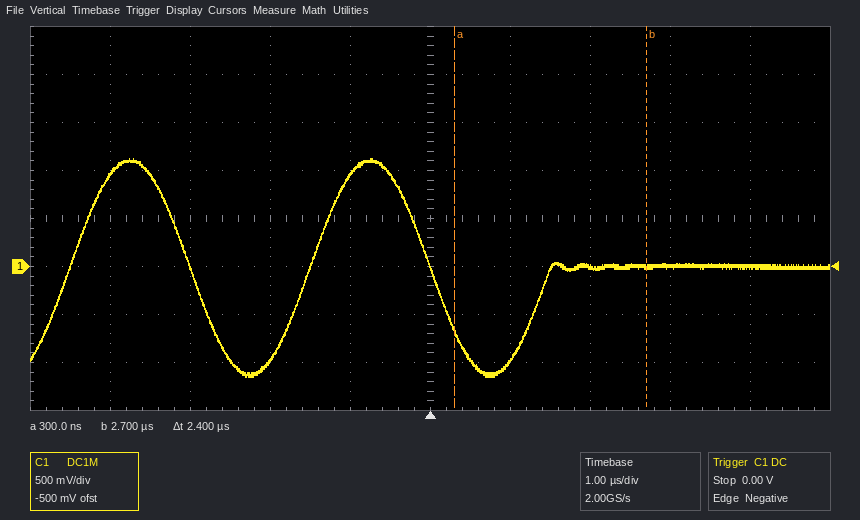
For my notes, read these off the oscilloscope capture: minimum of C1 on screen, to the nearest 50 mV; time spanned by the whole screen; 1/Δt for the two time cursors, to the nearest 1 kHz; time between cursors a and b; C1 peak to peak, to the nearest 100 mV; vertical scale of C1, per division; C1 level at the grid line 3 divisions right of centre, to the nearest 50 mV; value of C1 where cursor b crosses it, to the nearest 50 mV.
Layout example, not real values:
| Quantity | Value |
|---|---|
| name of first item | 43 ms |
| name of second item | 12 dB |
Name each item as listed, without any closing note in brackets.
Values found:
| Quantity | Value |
|---|---|
| minimum of C1 on screen, to the nearest 50 mV | -1.15 V |
| time spanned by the whole screen | 10 µs |
| 1/Δt for the two time cursors, to the nearest 1 kHz | 417 kHz |
| time between cursors a and b | 2.4 µs |
| C1 peak to peak, to the nearest 100 mV | 2.30 V |
| vertical scale of C1, per division | 500 mV |
| C1 level at the grid line 3 divisions right of centre, to the nearest 50 mV | 0 mV |
| value of C1 where cursor b crosses it, to the nearest 50 mV | 0 mV |
